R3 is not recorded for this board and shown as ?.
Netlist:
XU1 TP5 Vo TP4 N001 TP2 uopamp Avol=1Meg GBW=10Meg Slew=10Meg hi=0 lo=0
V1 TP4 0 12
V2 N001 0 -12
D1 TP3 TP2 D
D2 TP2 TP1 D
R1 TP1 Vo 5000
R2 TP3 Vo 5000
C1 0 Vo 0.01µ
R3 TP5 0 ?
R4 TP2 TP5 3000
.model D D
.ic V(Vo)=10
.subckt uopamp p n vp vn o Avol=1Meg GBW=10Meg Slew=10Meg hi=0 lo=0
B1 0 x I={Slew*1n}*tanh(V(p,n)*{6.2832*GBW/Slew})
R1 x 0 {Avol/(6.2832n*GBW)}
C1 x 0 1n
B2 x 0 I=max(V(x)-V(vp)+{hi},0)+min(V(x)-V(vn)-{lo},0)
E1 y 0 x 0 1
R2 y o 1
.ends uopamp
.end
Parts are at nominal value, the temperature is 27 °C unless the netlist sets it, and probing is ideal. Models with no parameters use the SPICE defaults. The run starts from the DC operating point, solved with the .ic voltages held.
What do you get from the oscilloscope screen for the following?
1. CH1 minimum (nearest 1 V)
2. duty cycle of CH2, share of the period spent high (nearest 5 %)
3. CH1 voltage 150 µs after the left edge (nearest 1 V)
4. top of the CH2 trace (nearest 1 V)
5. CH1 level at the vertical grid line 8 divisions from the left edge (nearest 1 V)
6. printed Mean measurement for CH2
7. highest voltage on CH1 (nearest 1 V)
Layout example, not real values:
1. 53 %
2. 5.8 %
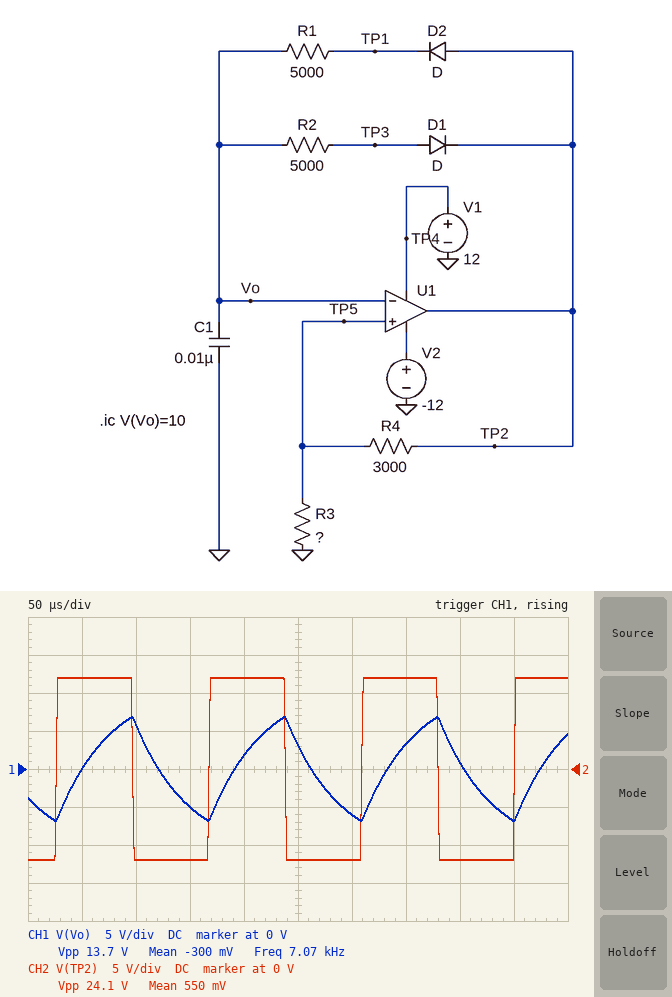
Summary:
1. -7 V
2. 50 %
3. -5 V
4. 12 V
5. 1 V
6. 550 mV
7. 7 V
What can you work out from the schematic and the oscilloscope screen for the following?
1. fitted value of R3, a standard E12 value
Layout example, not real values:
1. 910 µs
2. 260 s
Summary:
1. 3.9 kΩ
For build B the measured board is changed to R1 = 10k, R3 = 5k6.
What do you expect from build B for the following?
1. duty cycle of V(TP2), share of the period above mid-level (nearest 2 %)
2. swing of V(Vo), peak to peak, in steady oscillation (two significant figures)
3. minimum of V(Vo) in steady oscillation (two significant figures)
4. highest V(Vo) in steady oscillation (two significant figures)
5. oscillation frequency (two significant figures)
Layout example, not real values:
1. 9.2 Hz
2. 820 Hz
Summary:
1. 66 %
2. 16 V
3. -7.8 V
4. 7.8 V
5. 3.9 kHz
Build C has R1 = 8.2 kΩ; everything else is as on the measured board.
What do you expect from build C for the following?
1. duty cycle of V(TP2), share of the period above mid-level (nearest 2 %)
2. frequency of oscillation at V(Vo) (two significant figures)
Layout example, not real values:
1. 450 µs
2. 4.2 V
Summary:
1. 62 %
2. 5.4 kHz
